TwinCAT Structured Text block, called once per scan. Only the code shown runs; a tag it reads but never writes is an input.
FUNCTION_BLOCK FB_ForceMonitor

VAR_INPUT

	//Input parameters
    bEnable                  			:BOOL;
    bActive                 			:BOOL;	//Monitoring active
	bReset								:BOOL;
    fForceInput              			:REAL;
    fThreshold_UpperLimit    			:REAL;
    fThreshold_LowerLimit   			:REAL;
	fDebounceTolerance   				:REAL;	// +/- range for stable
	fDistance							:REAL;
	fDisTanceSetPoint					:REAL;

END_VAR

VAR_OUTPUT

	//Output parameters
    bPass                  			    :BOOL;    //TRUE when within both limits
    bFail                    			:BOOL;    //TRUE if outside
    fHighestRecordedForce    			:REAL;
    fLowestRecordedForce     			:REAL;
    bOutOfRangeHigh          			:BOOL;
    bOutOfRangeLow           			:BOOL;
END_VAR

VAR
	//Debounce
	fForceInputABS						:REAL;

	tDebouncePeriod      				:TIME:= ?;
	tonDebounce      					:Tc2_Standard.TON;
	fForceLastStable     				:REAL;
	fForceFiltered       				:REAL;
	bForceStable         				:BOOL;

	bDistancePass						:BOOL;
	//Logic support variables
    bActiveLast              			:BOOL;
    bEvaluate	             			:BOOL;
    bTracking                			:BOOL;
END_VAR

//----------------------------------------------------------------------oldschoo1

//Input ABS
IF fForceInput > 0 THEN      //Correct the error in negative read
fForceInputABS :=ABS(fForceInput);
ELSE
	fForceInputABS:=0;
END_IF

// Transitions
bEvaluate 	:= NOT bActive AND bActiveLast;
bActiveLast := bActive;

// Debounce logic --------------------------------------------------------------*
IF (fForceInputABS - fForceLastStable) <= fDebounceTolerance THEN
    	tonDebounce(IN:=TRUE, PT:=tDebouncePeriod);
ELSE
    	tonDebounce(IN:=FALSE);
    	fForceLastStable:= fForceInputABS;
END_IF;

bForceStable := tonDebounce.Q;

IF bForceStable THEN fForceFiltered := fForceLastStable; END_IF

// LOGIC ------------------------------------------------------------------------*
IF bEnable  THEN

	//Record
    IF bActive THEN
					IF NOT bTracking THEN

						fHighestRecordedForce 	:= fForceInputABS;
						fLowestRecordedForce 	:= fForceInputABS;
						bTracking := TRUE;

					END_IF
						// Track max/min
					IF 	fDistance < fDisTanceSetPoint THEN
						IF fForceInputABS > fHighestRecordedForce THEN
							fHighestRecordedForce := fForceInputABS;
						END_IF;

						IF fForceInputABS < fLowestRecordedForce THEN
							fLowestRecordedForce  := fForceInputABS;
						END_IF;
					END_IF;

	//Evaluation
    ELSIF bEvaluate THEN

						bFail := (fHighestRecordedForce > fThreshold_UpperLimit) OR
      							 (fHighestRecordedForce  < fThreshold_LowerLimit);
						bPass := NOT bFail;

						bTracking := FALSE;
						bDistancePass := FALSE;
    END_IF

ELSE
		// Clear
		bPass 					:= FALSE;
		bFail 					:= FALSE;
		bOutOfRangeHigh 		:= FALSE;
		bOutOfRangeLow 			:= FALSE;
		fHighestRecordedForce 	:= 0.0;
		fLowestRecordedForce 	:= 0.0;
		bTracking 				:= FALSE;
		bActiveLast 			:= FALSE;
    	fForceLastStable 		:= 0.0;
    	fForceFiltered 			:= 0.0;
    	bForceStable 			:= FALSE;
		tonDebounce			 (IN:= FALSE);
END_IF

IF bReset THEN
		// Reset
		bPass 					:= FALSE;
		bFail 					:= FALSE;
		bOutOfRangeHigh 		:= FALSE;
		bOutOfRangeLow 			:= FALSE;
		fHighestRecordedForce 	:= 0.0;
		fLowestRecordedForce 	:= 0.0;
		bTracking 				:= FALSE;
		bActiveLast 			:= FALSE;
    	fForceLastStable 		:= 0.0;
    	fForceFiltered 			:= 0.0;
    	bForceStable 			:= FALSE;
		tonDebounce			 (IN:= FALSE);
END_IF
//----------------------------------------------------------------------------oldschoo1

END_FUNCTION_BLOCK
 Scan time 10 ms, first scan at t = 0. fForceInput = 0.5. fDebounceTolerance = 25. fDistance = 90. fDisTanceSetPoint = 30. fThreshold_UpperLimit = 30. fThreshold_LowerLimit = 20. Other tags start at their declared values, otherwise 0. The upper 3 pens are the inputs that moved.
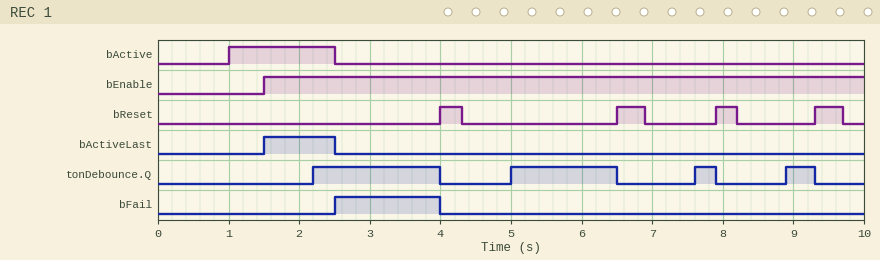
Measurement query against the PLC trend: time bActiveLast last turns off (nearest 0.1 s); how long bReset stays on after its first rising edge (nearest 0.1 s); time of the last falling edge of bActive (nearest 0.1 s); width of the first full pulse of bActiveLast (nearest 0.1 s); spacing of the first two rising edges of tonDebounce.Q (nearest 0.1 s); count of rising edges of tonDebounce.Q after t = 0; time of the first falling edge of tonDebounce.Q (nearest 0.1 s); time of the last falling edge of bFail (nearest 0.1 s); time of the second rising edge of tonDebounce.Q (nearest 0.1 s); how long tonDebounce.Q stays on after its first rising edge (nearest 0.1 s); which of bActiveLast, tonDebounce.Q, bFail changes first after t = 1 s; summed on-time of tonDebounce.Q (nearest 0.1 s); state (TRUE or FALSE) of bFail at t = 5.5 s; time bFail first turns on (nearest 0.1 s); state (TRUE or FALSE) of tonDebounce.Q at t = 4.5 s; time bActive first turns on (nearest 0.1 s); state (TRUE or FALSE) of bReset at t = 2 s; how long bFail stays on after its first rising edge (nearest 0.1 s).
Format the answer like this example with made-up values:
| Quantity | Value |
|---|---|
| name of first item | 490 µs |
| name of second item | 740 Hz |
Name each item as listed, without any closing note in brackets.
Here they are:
| Quantity | Value |
|---|---|
| time bActiveLast last turns off | 2.5 s |
| how long bReset stays on after its first rising edge | 0.3 s |
| time of the last falling edge of bActive | 2.5 s |
| width of the first full pulse of bActiveLast | 1.0 s |
| spacing of the first two rising edges of tonDebounce.Q | 2.8 s |
| count of rising edges of tonDebounce.Q after t = 0 | 4 |
| time of the first falling edge of tonDebounce.Q | 4.0 s |
| time of the last falling edge of bFail | 4.0 s |
| time of the second rising edge of tonDebounce.Q | 5.0 s |
| how long tonDebounce.Q stays on after its first rising edge | 1.8 s |
| which of bActiveLast, tonDebounce.Q, bFail changes first after t = 1 s | bActiveLast |
| summed on-time of tonDebounce.Q | 4.0 s |
| state (TRUE or FALSE) of bFail at t = 5.5 s | FALSE |
| time bFail first turns on | 2.5 s |
| state (TRUE or FALSE) of tonDebounce.Q at t = 4.5 s | FALSE |
| time bActive first turns on | 1.0 s |
| state (TRUE or FALSE) of bReset at t = 2 s | FALSE |
| how long bFail stays on after its first rising edge | 1.5 s |
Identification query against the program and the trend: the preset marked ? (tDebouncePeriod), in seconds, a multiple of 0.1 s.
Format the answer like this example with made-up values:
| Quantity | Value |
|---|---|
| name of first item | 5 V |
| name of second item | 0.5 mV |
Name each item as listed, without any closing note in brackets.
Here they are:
| Quantity | Value |
|---|---|
| the preset marked ? (tDebouncePeriod), in seconds, a multiple of 0.1 s | 0.7 s |
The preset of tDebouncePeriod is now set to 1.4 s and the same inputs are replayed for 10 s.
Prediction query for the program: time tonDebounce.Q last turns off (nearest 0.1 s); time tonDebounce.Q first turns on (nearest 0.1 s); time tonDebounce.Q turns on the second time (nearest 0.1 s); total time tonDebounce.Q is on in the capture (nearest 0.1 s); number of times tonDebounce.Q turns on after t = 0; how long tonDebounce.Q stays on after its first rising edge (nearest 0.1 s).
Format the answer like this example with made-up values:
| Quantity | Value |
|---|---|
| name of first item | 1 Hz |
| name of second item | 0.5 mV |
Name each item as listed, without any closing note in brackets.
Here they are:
| Quantity | Value |
|---|---|
| time tonDebounce.Q last turns off | 6.5 s |
| time tonDebounce.Q first turns on | 2.9 s |
| time tonDebounce.Q turns on the second time | 5.7 s |
| total time tonDebounce.Q is on in the capture | 1.9 s |
| number of times tonDebounce.Q turns on after t = 0 | 2 |
| how long tonDebounce.Q stays on after its first rising edge | 1.1 s |
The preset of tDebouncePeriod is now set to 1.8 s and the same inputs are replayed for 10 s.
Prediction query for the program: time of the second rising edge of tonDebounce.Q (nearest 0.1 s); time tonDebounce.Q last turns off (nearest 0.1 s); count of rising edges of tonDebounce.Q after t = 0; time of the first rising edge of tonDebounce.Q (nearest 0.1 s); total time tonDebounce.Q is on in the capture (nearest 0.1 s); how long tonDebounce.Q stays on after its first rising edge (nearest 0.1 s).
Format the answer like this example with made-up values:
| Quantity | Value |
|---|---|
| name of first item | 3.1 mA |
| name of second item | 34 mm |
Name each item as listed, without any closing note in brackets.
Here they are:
| Quantity | Value |
|---|---|
| time of the second rising edge of tonDebounce.Q | 6.1 s |
| time tonDebounce.Q last turns off | 6.5 s |
| count of rising edges of tonDebounce.Q after t = 0 | 2 |
| time of the first rising edge of tonDebounce.Q | 3.3 s |
| total time tonDebounce.Q is on in the capture | 1.1 s |
| how long tonDebounce.Q stays on after its first rising edge | 0.7 s |
